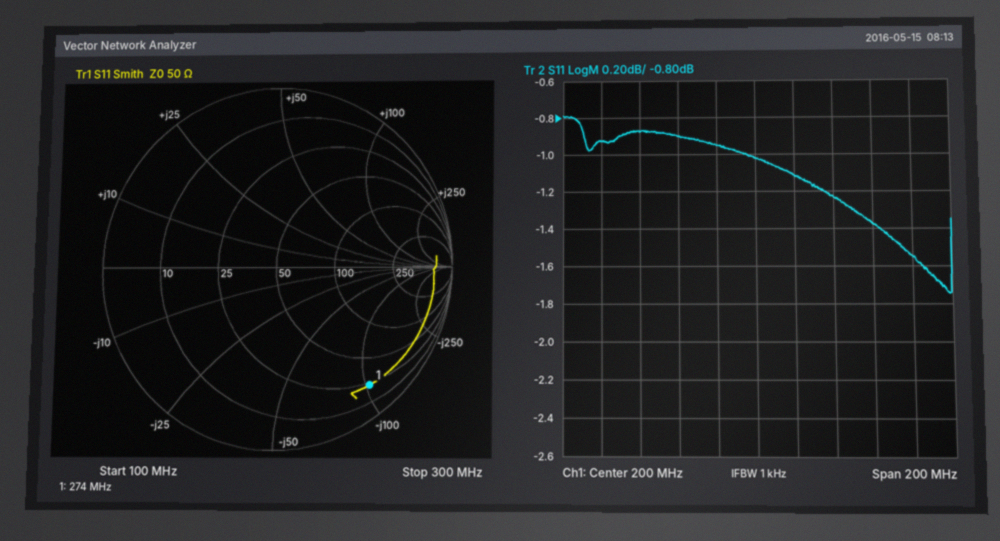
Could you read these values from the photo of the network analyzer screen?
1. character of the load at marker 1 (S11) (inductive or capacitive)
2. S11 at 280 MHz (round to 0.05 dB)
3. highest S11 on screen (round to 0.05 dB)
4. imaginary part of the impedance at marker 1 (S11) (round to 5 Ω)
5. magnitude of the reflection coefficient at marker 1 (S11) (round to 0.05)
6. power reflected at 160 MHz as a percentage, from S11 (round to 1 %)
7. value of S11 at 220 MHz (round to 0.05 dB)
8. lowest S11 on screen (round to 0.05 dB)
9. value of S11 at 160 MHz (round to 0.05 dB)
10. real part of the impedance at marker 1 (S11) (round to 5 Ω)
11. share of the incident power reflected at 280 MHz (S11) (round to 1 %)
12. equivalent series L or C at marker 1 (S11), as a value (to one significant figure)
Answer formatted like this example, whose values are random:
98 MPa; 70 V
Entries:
capacitive; -1.55 dB; -0.80 dB; -105 Ω; 0.85; 81 %; -1.10 dB; -1.75 dB; -0.90 dB; 25 Ω; 70 %; 6 pF
